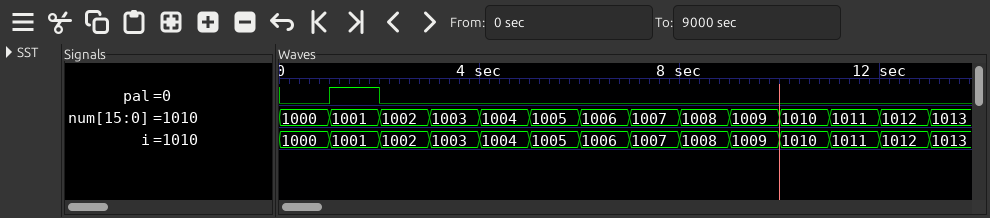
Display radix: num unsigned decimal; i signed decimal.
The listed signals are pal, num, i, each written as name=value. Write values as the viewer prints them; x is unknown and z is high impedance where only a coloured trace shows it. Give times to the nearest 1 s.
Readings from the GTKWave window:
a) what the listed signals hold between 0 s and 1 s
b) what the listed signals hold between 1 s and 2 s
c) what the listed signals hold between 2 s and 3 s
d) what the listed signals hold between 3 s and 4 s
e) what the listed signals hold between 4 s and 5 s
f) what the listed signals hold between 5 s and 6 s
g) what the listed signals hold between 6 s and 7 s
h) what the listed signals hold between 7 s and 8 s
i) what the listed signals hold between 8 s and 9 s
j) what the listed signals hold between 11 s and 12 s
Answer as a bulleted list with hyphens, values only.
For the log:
- pal=0, num=1000, i=1000
- pal=1, num=1001, i=1001
- pal=0, num=1002, i=1002
- pal=0, num=1003, i=1003
- pal=0, num=1004, i=1004
- pal=0, num=1005, i=1005
- pal=0, num=1006, i=1006
- pal=0, num=1007, i=1007
- pal=0, num=1008, i=1008
- pal=0, num=1011, i=1011
